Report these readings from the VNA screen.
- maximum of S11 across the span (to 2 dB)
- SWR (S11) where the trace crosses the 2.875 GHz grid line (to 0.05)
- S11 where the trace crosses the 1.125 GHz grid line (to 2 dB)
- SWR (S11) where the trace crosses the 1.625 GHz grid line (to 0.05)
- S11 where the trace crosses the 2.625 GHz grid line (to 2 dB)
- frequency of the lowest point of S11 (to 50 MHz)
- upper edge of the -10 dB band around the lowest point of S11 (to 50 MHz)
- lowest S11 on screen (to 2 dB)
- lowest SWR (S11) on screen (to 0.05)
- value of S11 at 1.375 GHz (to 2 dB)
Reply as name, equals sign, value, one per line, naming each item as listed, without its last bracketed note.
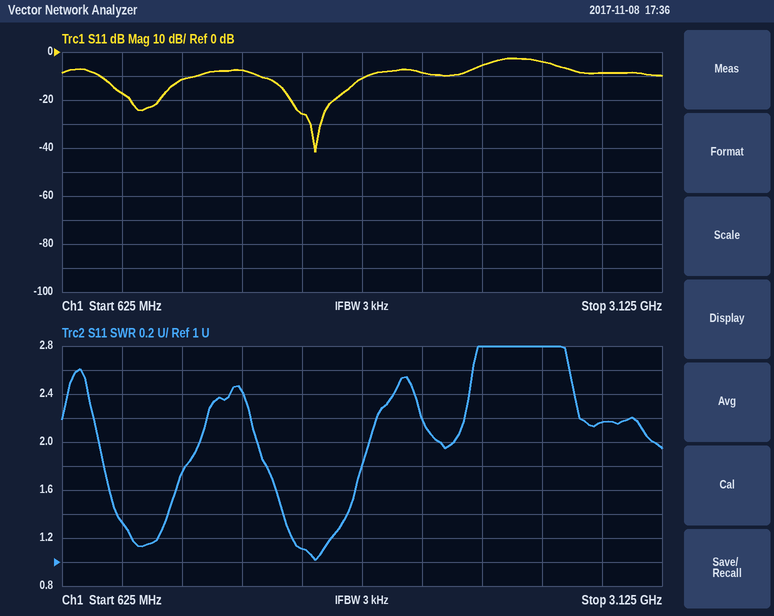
maximum of S11 across the span = -2 dB
SWR (S11) where the trace crosses the 2.875 GHz grid line = 2.15
S11 where the trace crosses the 1.125 GHz grid line = -12 dB
SWR (S11) where the trace crosses the 1.625 GHz grid line = 1.10
S11 where the trace crosses the 2.625 GHz grid line = -4 dB
frequency of the lowest point of S11 = 1.70 GHz
upper edge of the -10 dB band around the lowest point of S11 = 1.90 GHz
lowest S11 on screen = -42 dB
lowest SWR (S11) on screen = 1.00
value of S11 at 1.375 GHz = -8 dB
